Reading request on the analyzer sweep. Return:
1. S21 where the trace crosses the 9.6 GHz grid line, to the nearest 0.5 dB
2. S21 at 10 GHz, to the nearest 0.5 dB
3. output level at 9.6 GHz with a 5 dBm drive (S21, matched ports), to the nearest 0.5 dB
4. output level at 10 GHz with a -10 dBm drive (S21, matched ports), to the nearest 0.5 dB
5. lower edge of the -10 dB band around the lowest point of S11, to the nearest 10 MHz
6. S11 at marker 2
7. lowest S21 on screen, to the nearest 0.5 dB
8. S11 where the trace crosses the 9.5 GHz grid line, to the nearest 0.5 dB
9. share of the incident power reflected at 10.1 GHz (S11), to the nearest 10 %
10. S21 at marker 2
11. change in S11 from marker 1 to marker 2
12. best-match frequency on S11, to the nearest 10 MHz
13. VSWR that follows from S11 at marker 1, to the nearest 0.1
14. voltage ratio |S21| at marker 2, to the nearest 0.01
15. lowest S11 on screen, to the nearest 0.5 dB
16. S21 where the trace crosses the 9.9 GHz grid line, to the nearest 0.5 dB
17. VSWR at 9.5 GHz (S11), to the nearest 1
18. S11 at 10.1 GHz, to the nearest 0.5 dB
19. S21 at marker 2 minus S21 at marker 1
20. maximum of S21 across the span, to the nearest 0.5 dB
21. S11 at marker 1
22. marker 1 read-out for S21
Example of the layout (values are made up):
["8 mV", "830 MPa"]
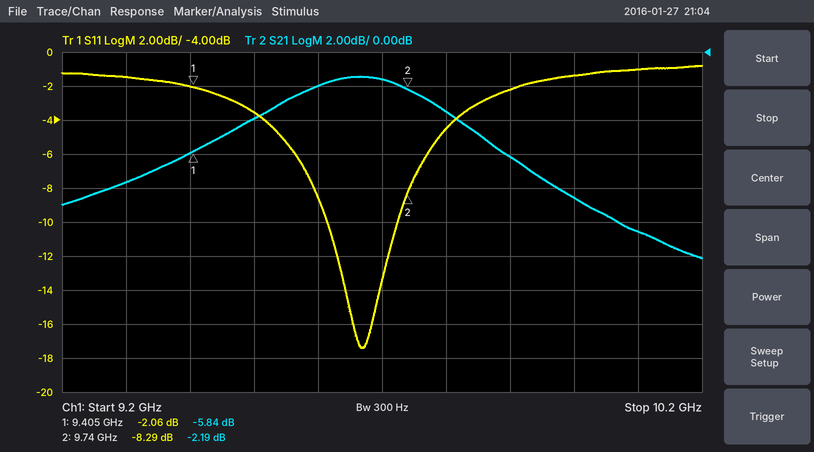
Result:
["-2.0 dB", "-8.5 dB", "3.0 dBm", "-18.5 dBm", "9.61 GHz", "-8.29 dB", "-12.0 dB", "-3.5 dB", "80 %", "-2.19 dB", "-6.23 dB", "9.67 GHz", "8.5", "0.78", "-17.5 dB", "-6.0 dB", "5", "-1.0 dB", "3.65 dB", "-1.5 dB", "-2.06 dB", "-5.84 dB"]
